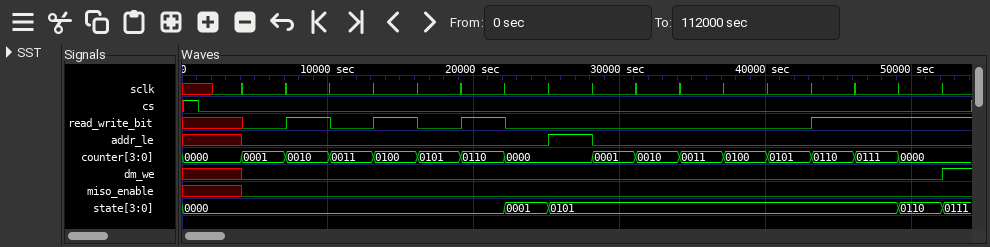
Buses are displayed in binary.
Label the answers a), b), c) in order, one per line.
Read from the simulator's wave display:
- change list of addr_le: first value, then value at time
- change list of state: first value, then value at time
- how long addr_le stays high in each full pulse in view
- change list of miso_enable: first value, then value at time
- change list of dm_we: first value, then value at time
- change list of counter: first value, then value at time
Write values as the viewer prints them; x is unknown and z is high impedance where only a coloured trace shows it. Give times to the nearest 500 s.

a) x, 0 at 4000 s, 1 at 25000 s, 0 at 28000 s
b) 0000, 0001 at 22000 s, 0101 at 25000 s, 0110 at 49000 s, 0111 at 52000 s
c) 3000 s
d) x, 0 at 4000 s
e) x, 0 at 4000 s, 1 at 52000 s
f) 0000, 0001 at 4000 s, 0010 at 7000 s, 0011 at 10000 s, 0100 at 13000 s, 0101 at 16000 s, 0110 at 19000 s, 0000 at 22000 s, 0001 at 28000 s, 0010 at 31000 s, 0011 at 34000 s, 0100 at 37000 s, 0101 at 40000 s, 0110 at 43000 s, 0111 at 46000 s, 0000 at 49000 s
